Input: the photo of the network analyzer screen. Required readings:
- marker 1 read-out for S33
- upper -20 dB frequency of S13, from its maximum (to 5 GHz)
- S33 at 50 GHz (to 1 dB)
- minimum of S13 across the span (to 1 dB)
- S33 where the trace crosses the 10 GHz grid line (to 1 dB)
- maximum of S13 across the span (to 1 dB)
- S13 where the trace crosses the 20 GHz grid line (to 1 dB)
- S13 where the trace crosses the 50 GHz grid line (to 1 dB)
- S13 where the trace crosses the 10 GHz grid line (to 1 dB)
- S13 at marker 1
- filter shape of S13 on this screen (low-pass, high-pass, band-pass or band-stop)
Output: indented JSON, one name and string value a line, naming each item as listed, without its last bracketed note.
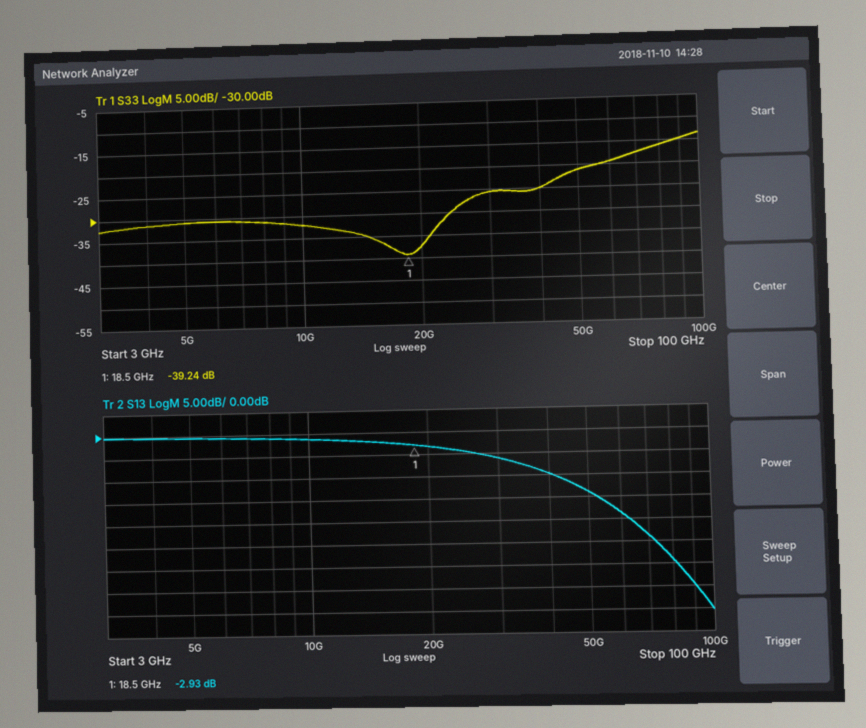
{
  "marker 1 read-out for S33": "-39.24 dB",
  "upper -20 dB frequency of S13, from its maximum": "65 GHz",
  "S33 at 50 GHz": "-21 dB",
  "minimum of S13 across the span": "-40 dB",
  "S33 where the trace crosses the 10 GHz grid line": "-32 dB",
  "maximum of S13 across the span": "0 dB",
  "S13 where the trace crosses the 20 GHz grid line": "-3 dB",
  "S13 where the trace crosses the 50 GHz grid line": "-14 dB",
  "S13 where the trace crosses the 10 GHz grid line": "-1 dB",
  "S13 at marker 1": "-2.93 dB",
  "filter shape of S13 on this screen": "low-pass"
}
